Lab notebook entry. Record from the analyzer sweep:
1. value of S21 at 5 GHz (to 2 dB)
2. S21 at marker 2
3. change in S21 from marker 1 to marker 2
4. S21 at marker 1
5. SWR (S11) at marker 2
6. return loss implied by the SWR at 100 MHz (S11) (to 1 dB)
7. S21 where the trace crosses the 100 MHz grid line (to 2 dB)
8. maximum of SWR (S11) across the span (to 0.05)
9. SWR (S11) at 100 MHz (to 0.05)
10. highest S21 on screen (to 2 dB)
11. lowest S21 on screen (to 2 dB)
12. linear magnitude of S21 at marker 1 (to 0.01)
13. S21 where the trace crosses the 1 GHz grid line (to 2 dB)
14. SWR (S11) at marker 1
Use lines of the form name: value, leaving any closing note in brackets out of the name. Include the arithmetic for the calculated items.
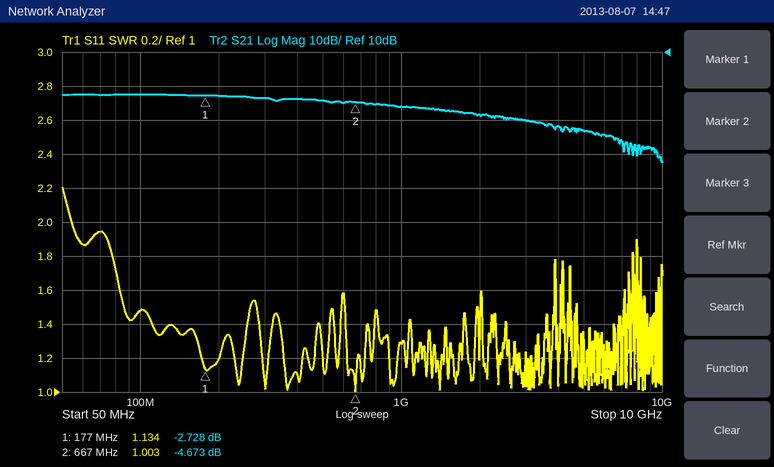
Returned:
value of S21 at 5 GHz: -14 dB
S21 at marker 2: -4.673 dB
change in S21 from marker 1 to marker 2: -4.673 − (-2.728) = -1.945 dB
S21 at marker 1: -2.728 dB
SWR (S11) at marker 2: 1.003
return loss implied by the SWR at 100 MHz (S11): −20 log10((1.5 − 1)/(1.5 + 1)) ≈ 14 dB
S21 where the trace crosses the 100 MHz grid line: -2 dB
maximum of SWR (S11) across the span: 2.20
SWR (S11) at 100 MHz: 1.50
highest S21 on screen: -2 dB
lowest S21 on screen: -22 dB
linear magnitude of S21 at marker 1: 10^(-2.728/20) ≈ 0.73
S21 where the trace crosses the 1 GHz grid line: -6 dB
SWR (S11) at marker 1: 1.134
